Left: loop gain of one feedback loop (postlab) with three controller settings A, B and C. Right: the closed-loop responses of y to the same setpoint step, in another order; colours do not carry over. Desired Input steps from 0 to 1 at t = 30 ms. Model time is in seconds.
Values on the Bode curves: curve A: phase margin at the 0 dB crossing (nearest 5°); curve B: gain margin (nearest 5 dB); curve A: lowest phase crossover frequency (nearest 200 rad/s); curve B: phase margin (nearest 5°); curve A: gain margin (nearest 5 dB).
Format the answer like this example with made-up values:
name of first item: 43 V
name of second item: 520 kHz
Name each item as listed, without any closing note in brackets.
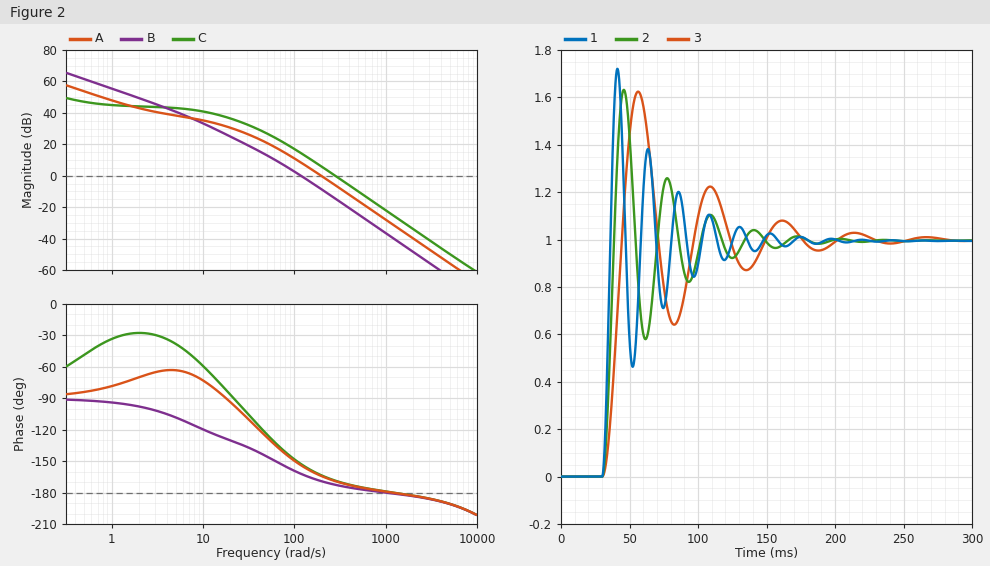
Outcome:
curve A: phase margin at the 0 dB crossing: 15°
curve B: gain margin: 35 dB
curve A: lowest phase crossover frequency: 1200 rad/s
curve B: phase margin: 20°
curve A: gain margin: 30 dB
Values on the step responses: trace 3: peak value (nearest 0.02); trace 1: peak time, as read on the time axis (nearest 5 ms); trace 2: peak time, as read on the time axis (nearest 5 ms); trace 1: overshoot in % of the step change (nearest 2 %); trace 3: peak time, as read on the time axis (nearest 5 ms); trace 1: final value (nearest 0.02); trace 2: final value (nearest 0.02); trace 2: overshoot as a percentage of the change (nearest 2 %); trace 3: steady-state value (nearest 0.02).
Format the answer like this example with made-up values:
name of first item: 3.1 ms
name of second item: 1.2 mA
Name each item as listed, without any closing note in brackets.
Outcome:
trace 3: peak value: 1.62
trace 1: peak time, as read on the time axis: 40 ms
trace 2: peak time, as read on the time axis: 45 ms
trace 1: overshoot in % of the step change: 72 %
trace 3: peak time, as read on the time axis: 55 ms
trace 1: final value: 1.00
trace 2: final value: 1.00
trace 2: overshoot as a percentage of the change: 64 %
trace 3: steady-state value: 1.00
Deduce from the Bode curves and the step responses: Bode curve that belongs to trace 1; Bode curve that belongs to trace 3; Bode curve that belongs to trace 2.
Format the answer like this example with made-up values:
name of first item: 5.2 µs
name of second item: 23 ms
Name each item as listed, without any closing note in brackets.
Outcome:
Bode curve that belongs to trace 1: C
Bode curve that belongs to trace 3: B
Bode curve that belongs to trace 2: A
